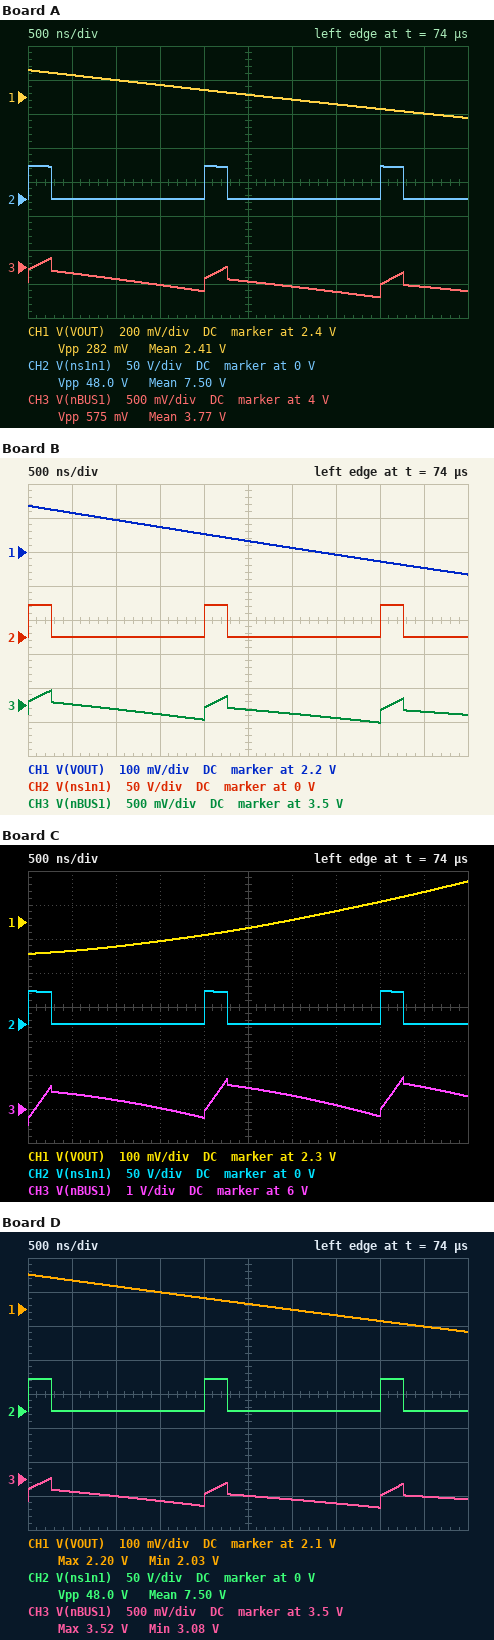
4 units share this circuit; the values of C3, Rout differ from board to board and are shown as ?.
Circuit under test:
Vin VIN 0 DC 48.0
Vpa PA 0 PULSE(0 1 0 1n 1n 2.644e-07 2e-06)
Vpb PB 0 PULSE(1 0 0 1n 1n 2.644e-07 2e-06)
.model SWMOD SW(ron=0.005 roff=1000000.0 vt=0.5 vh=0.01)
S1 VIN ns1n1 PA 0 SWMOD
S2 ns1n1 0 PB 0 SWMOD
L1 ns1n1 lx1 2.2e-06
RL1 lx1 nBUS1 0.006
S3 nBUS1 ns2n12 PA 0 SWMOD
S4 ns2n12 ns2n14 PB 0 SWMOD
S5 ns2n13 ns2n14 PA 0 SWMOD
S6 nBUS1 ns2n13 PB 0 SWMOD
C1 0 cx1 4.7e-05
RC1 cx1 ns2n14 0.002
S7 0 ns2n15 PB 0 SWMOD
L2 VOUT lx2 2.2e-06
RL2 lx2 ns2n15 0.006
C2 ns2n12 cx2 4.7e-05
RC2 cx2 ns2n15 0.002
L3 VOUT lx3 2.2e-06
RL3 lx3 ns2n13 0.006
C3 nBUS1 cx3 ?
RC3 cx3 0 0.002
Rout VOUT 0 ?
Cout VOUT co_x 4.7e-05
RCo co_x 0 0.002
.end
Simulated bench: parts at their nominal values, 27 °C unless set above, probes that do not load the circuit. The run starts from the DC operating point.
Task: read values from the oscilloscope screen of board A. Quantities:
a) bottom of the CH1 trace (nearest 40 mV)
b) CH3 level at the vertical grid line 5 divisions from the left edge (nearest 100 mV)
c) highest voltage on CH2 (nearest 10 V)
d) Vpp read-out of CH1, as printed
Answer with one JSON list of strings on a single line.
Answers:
["2.28 V", "3.8 V", "50 V", "282 mV"]
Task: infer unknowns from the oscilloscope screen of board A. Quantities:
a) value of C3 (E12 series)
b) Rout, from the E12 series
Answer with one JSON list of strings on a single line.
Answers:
["120 µF", "0.082 Ω"]
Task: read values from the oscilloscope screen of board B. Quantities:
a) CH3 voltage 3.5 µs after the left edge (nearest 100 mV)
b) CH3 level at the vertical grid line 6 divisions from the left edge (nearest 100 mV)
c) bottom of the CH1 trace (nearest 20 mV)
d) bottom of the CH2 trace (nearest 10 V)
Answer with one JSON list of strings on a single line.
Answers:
["3.3 V", "3.4 V", "2.14 V", "0 V"]
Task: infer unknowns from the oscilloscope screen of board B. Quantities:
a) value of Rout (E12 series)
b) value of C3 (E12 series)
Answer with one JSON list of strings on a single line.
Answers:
["0.056 Ω", "120 µF"]
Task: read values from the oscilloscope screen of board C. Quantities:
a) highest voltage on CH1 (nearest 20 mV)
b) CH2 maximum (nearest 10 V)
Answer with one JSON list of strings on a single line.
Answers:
["2.42 V", "50 V"]
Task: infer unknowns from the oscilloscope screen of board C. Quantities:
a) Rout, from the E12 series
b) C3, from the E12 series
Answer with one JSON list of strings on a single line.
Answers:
["0.18 Ω", "22 µF"]
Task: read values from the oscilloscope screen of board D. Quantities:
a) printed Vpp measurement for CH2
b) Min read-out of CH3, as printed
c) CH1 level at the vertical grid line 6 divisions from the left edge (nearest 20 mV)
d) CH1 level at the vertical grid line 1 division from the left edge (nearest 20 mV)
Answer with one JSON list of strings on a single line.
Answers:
["48.0 V", "3.08 V", "2.10 V", "2.18 V"]
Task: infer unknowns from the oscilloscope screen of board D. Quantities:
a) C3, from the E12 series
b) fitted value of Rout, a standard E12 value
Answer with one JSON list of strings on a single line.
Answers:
["120 µF", "0.047 Ω"]
